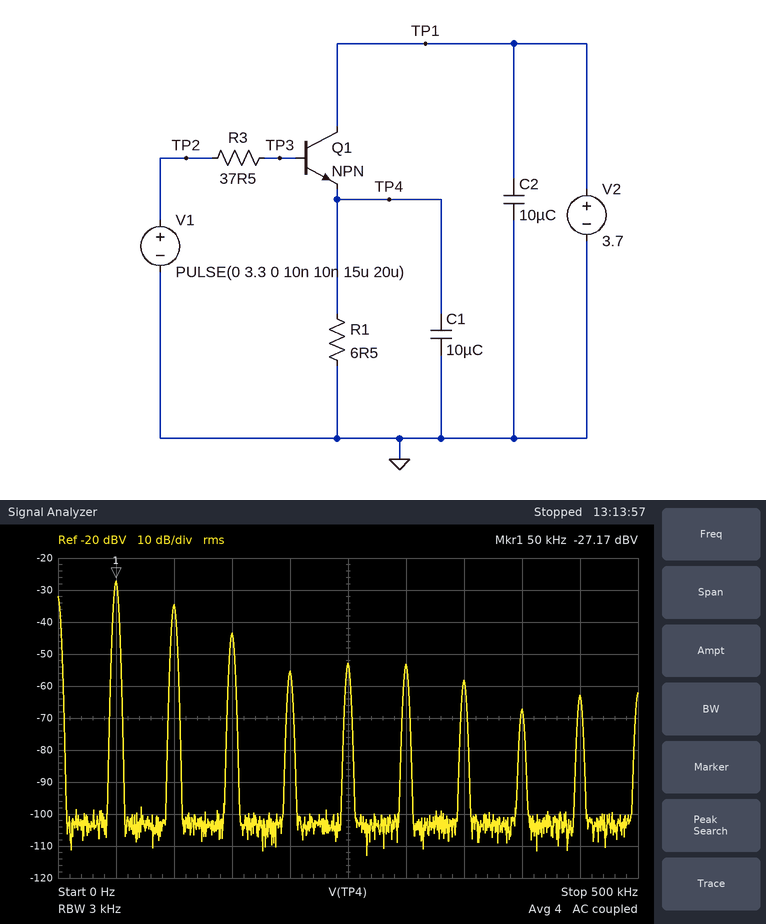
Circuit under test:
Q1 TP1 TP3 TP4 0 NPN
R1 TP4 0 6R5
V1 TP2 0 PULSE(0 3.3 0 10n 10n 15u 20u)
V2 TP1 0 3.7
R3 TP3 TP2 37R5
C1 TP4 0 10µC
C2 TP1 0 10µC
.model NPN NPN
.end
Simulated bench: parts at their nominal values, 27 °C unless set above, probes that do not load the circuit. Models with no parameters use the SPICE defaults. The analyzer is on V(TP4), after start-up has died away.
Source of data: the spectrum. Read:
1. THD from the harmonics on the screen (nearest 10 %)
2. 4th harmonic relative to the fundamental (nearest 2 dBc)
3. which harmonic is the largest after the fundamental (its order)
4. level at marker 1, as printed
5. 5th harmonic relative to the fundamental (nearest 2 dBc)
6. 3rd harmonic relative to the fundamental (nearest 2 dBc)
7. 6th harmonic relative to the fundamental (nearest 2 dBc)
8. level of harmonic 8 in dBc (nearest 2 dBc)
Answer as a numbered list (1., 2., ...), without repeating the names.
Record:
1. 50 %
2. -28 dBc
3. 2
4. -27.17 dBV
5. -26 dBc
6. -16 dBc
7. -26 dBc
8. -40 dBc
